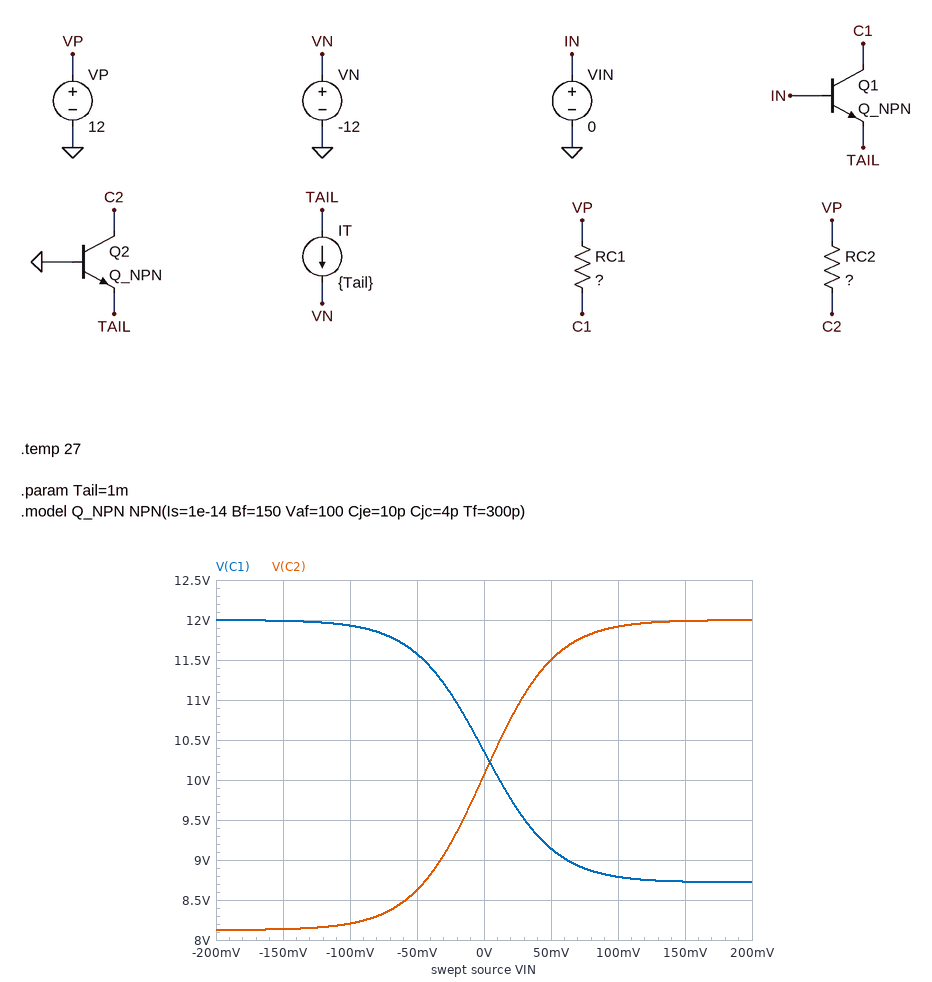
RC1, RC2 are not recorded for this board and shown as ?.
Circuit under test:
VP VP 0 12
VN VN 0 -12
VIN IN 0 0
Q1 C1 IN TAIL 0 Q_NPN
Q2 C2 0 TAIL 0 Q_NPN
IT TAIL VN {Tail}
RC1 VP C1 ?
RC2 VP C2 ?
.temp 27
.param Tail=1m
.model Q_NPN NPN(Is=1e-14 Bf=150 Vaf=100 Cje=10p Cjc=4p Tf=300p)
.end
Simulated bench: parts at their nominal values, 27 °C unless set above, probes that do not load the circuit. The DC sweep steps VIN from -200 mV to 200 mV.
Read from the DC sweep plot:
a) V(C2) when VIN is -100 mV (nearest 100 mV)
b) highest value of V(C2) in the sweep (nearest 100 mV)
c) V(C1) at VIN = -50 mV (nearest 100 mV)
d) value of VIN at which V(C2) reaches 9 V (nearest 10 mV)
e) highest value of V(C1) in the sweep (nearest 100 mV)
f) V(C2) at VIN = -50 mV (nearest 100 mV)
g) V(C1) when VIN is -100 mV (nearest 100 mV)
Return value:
8.2 V
12.0 V
11.6 V
-30 mV
12.0 V
8.6 V
11.9 V
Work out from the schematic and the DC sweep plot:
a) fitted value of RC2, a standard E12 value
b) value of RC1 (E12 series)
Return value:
3.9 kΩ
3.3 kΩ
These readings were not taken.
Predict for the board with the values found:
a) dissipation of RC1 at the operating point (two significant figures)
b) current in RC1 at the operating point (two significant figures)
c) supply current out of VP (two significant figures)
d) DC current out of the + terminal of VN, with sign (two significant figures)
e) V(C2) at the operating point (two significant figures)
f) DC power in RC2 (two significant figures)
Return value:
820 µW
500 µA
990 µA
-1.0 mA
10 V
960 µW
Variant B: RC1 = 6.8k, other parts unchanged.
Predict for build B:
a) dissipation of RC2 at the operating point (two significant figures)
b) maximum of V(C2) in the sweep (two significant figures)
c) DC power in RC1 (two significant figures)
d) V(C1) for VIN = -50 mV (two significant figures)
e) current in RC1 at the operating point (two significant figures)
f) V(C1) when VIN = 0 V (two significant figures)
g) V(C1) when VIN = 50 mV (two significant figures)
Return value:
980 µW
12 V
1.7 mW
11 V
490 µA
8.6 V
6.1 V
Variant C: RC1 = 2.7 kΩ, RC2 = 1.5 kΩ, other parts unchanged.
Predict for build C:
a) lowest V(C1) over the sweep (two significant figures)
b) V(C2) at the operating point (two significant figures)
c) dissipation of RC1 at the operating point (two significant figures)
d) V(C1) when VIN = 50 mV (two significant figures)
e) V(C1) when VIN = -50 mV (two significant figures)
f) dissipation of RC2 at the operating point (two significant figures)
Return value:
9.3 V
11 V
660 µW
9.7 V
12 V
370 µW
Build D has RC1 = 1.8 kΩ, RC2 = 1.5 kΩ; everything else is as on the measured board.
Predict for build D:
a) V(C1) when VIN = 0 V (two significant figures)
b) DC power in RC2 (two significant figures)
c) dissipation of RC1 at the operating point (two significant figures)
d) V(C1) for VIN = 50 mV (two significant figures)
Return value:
11 V
370 µW
440 µW
10 V
